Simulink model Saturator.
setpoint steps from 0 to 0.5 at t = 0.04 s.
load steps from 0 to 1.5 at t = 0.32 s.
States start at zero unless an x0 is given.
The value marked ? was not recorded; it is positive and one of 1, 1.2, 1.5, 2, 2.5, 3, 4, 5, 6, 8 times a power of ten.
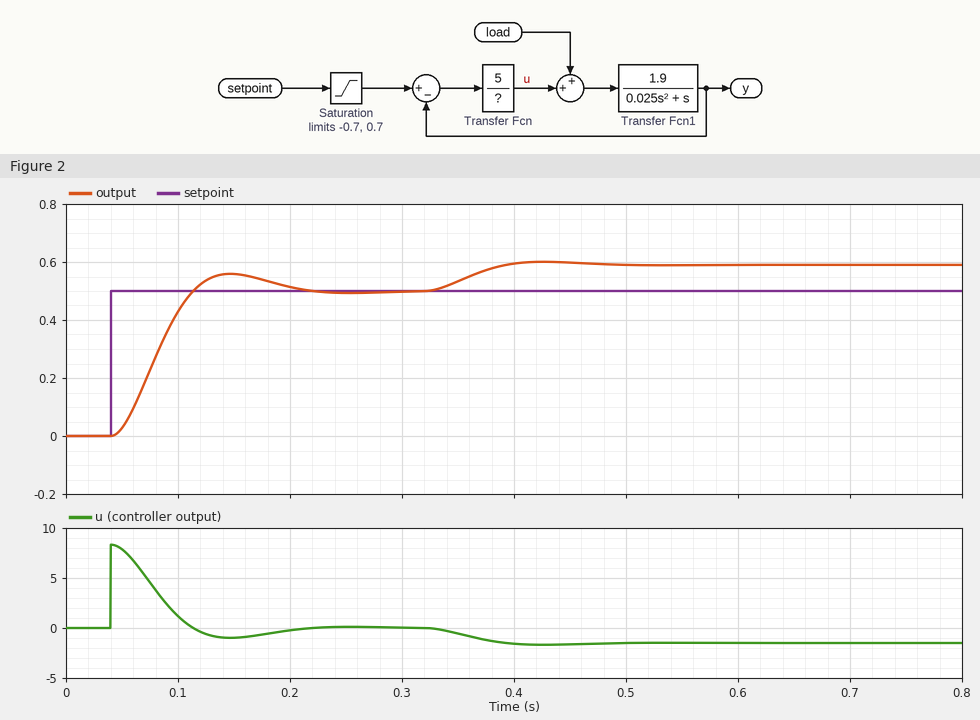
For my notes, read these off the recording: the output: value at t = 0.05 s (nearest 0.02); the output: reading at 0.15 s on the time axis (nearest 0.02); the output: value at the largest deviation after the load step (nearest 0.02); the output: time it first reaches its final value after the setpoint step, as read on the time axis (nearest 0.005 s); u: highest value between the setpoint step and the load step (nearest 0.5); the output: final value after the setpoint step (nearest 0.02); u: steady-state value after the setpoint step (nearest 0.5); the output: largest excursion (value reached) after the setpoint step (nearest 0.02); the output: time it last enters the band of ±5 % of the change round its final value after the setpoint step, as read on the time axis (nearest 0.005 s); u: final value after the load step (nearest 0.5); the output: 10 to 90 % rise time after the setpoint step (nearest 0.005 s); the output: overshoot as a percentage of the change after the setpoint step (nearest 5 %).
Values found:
0.02
0.56
0.60
0.115 s
8.5
0.50
0.0
0.56
0.190 s
-1.5
0.050 s
10 %
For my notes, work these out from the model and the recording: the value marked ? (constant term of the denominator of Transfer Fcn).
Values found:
0.3
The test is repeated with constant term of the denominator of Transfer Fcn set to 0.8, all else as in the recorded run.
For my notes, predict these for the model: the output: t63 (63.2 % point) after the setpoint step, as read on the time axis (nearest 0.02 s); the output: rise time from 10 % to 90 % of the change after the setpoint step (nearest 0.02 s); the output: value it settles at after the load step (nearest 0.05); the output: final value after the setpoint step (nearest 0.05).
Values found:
0.14 s
0.14 s
0.75
0.50
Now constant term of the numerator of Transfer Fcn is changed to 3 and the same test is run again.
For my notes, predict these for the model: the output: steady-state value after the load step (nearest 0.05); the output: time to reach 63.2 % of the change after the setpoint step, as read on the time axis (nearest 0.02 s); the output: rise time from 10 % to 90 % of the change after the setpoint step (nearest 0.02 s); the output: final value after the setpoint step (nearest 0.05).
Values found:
0.65
0.10 s
0.08 s
0.50
